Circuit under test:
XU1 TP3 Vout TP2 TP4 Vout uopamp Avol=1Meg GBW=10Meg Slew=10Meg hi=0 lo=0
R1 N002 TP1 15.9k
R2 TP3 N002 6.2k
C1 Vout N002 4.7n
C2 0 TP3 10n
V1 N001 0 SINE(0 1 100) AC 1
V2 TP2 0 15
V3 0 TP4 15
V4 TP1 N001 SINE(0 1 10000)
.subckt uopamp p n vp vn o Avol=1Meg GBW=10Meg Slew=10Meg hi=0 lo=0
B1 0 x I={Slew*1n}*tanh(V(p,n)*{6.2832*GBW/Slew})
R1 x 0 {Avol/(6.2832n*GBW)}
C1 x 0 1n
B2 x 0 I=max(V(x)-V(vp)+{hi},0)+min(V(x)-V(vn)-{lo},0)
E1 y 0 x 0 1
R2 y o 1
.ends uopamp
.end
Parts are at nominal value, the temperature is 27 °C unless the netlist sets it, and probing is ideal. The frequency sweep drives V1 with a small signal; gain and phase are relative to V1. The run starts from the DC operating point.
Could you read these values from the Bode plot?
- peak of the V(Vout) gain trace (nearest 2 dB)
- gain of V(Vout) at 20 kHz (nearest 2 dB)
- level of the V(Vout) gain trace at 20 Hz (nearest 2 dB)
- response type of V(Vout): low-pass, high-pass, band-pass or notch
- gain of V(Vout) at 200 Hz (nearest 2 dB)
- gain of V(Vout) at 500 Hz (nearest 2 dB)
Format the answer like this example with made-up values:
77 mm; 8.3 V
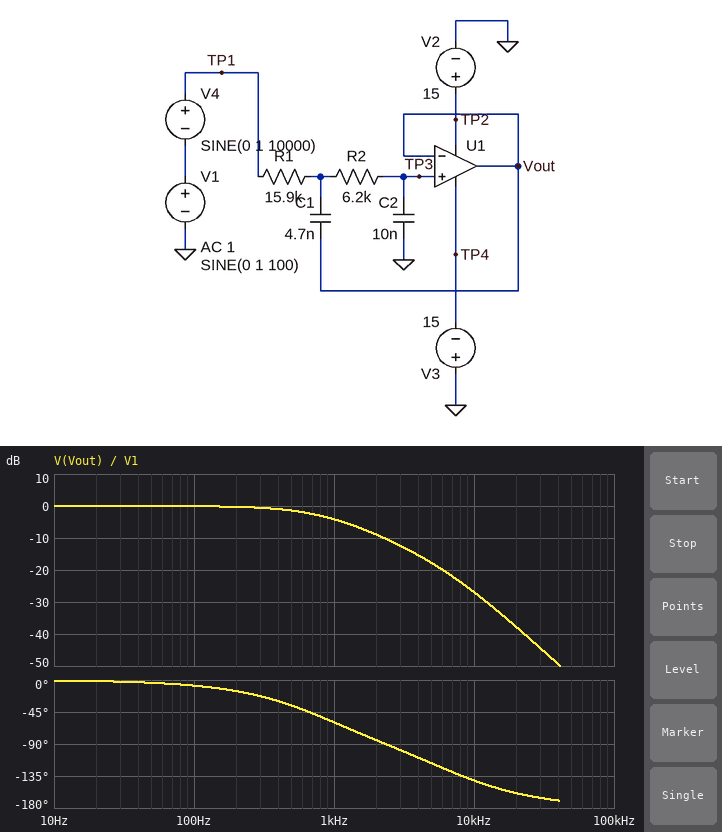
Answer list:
0 dB; -38 dB; 0 dB; low-pass; 0 dB; -2 dB
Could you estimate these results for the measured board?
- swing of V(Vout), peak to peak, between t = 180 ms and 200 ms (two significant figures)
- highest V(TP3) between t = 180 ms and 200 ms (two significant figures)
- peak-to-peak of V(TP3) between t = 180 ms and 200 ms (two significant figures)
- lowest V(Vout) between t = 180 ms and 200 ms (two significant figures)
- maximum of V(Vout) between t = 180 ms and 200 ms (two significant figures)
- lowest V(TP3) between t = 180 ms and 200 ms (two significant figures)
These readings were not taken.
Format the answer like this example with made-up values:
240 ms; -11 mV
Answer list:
2.1 V; 1.0 V; 2.1 V; -1.0 V; 1.0 V; -1.0 V
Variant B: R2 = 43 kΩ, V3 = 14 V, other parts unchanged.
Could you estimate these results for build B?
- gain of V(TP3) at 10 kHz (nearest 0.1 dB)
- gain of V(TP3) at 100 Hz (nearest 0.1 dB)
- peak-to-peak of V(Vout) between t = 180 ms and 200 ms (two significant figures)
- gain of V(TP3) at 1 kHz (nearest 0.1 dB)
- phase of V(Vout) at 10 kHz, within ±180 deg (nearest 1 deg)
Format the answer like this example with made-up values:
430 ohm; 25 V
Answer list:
-42.4 dB; -0.5 dB; 1.9 V; -11.4 dB; -164 deg
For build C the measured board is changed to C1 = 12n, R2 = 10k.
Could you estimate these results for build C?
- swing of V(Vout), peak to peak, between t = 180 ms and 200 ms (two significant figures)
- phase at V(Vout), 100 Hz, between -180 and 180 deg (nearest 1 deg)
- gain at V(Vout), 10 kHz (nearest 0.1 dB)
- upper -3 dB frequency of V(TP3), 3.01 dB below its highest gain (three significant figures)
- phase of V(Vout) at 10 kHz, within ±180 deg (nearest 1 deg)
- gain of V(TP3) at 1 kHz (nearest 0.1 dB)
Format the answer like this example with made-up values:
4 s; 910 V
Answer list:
2.0 V; -9 deg; -37.6 dB; 812 Hz; -168 deg; -4.3 dB
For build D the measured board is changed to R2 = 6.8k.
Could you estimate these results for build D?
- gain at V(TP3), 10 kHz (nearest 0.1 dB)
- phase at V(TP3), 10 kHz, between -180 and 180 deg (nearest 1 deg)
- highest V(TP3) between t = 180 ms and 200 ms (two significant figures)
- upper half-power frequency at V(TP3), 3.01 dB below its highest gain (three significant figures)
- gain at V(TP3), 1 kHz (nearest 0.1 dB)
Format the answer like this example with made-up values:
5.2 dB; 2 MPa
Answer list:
-27.5 dB; -143 deg; 1.0 V; 777 Hz; -4.3 dB
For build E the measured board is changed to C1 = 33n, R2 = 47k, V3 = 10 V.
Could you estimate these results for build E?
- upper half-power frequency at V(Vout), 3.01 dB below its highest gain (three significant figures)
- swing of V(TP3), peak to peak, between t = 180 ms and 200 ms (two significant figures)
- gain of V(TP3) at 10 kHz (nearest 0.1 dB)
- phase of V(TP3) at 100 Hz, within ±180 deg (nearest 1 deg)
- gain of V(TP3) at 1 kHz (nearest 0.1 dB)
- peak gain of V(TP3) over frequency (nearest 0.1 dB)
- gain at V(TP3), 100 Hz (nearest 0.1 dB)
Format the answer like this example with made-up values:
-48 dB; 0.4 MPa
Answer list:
348 Hz; 2.0 V; -59.8 dB; -24 deg; -19.6 dB; 0.2 dB; 0.1 dB
